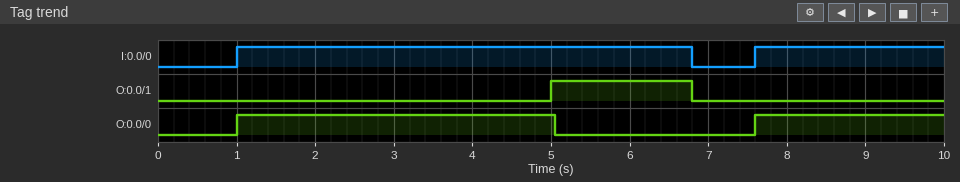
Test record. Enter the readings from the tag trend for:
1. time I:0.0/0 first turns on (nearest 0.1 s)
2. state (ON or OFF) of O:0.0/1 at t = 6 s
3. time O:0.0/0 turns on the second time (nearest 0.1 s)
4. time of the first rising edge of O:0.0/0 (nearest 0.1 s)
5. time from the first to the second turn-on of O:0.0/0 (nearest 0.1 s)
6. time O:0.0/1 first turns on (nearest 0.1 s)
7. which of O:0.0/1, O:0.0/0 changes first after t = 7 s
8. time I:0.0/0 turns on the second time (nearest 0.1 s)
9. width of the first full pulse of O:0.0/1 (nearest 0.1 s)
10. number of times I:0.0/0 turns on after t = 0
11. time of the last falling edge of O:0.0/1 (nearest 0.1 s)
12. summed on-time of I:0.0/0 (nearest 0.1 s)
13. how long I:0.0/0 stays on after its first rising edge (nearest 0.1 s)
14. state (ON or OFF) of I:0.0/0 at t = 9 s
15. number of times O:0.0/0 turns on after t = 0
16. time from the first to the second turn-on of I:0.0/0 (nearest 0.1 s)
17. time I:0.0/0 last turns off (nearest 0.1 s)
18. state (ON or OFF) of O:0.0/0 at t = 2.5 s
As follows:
1.0 s
ON
7.6 s
1.0 s
6.6 s
5.0 s
O:0.0/0
7.6 s
1.8 s
2
6.8 s
8.2 s
5.8 s
ON
2
6.6 s
6.8 s
ON
